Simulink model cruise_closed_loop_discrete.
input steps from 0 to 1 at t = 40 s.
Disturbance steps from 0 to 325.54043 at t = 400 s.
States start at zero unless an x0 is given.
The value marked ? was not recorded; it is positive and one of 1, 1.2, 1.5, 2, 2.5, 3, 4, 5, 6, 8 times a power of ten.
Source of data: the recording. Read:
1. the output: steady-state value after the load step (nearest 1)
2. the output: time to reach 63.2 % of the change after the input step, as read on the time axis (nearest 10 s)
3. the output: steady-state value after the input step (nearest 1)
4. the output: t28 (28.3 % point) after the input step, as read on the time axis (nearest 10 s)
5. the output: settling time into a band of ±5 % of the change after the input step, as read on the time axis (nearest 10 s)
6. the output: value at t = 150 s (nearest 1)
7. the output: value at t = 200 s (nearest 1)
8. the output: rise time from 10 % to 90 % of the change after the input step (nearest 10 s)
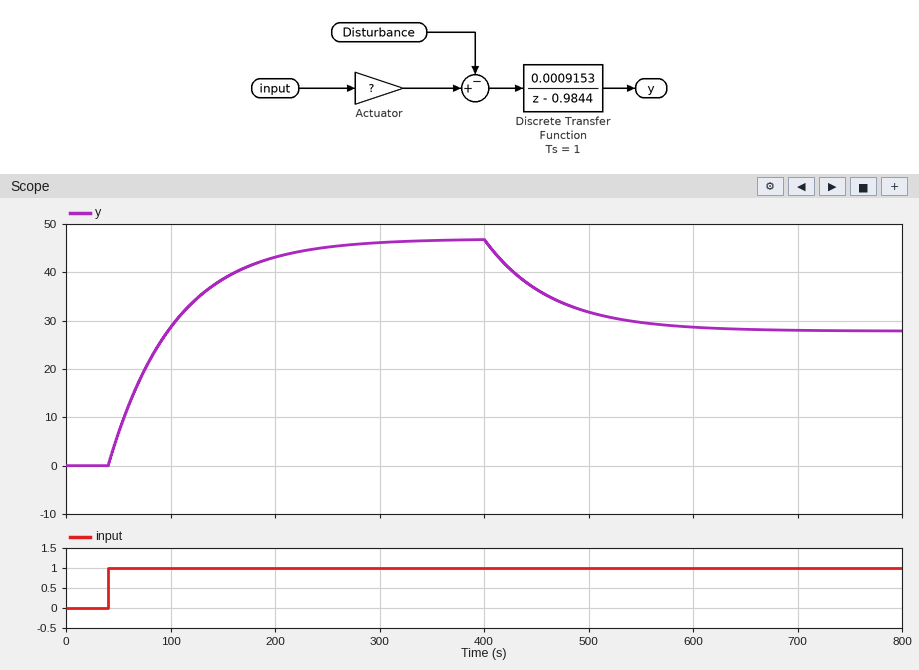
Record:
28
100 s
47
60 s
230 s
39
43
140 s
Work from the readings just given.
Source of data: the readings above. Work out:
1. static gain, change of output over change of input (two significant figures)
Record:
47
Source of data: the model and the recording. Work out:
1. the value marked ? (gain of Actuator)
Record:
800
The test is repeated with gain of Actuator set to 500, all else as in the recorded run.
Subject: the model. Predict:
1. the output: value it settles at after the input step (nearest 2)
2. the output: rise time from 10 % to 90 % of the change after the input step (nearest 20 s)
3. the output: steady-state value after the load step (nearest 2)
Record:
30
140 s
10
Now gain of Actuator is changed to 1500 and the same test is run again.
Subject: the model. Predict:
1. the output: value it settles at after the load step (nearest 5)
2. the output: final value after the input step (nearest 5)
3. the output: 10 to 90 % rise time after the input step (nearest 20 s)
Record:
70
90
140 s
